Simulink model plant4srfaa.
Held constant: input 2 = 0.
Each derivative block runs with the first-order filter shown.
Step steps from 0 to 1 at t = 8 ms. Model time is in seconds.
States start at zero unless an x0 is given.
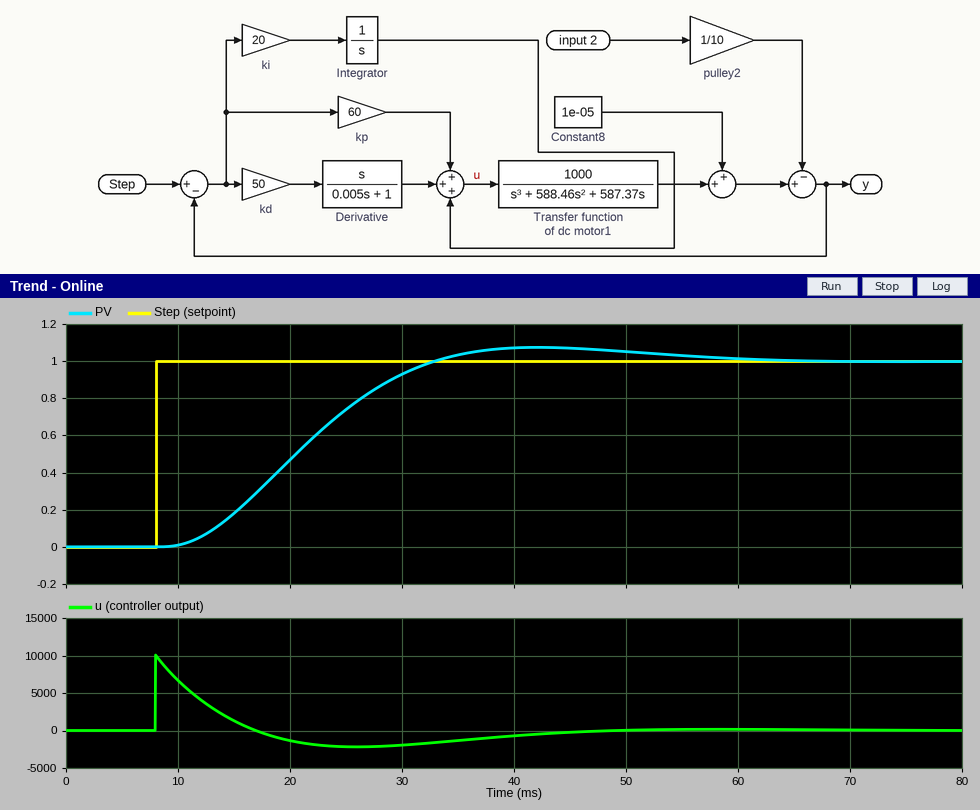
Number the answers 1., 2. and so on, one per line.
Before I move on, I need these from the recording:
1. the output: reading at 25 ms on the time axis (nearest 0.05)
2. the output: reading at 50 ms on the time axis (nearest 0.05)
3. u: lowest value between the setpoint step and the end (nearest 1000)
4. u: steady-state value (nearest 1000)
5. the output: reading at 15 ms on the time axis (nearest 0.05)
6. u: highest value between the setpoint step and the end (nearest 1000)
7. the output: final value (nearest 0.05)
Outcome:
1. 0.75
2. 1.05
3. -2000
4. 0
5. 0.20
6. 10000
7. 1.00
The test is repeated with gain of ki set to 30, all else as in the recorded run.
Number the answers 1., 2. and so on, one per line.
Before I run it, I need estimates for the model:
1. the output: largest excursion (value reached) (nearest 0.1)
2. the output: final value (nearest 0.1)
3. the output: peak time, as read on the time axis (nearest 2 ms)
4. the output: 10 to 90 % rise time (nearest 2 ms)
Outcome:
1. 1.1
2. 1.0
3. 42 ms
4. 16 ms
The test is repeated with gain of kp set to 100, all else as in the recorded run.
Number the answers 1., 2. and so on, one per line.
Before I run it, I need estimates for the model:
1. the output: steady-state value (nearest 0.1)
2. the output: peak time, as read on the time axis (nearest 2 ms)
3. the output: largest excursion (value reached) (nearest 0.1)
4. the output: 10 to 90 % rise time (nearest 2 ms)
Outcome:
1. 1.0
2. 42 ms
3. 1.1
4. 16 ms
